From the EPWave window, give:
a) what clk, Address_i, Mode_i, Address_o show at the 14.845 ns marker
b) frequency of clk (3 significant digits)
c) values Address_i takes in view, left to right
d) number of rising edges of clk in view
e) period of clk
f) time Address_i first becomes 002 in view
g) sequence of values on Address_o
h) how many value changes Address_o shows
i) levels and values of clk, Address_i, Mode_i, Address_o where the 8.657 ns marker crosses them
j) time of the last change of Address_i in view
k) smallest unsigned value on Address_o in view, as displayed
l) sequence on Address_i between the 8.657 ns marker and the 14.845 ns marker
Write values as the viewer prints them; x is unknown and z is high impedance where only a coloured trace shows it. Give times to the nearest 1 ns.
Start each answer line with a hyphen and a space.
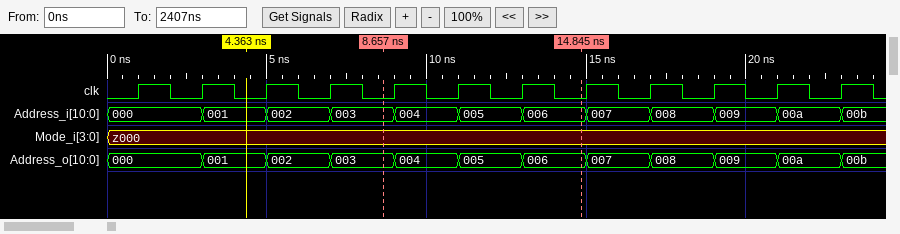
- clk=0, Address_i=006, Mode_i=z000, Address_o=006
- 500 MHz
- 000, 001, 002, 003, 004, 005, 006, 007, 008, 009, 00a, 00b
- 12
- 2 ns
- 5 ns
- 000, 001, 002, 003, 004, 005, 006, 007, 008, 009, 00a, 00b
- 11
- clk=0, Address_i=003, Mode_i=z000, Address_o=003
- 23 ns
- 000
- 003, 004, 005, 006
